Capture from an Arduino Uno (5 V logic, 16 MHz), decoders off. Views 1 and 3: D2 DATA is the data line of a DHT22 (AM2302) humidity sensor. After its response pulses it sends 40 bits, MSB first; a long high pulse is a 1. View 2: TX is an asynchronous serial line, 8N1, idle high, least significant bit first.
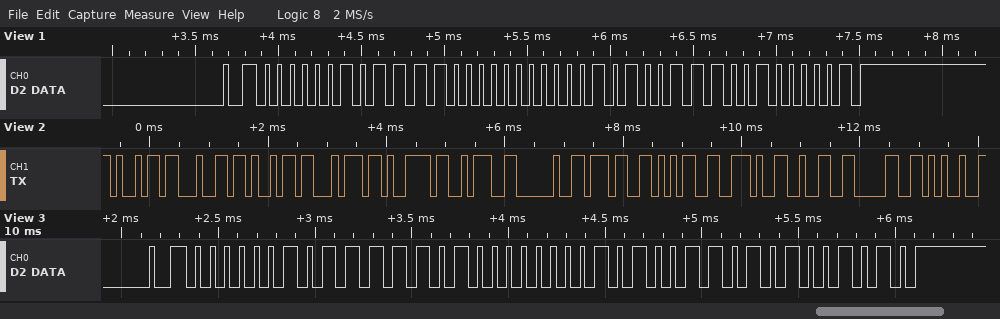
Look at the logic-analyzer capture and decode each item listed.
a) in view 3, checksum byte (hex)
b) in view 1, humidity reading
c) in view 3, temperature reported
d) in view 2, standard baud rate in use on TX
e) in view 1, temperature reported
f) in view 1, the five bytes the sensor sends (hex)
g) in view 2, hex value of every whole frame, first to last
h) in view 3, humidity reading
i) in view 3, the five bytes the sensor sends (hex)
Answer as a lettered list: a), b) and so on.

a) 0x4A
b) 75.2 %
c) 33.3 °C
d) 9600 baud
e) 33.4 °C
f) 02 F0 01 4E 41
g) 0x69 0x64 0x69 0x74 0x79 0x3A 0x20 0x37 0x35 0x2E 0x32 0x30 0x25
h) 76.2 %
i) 02 FA 01 4D 4A
